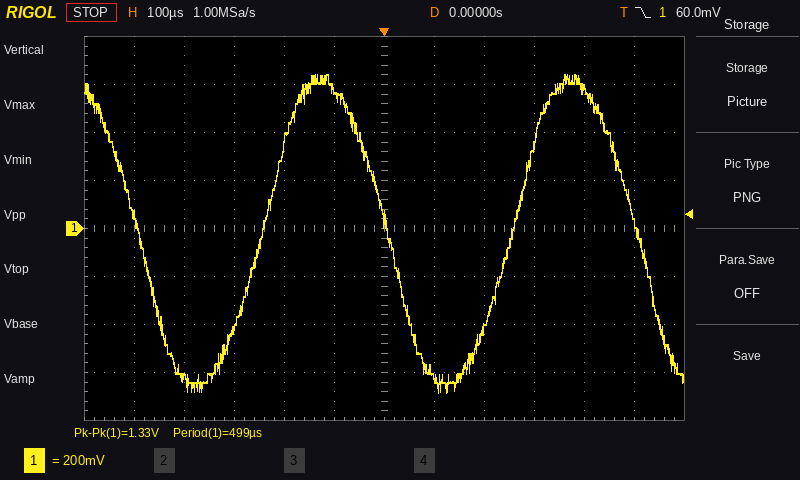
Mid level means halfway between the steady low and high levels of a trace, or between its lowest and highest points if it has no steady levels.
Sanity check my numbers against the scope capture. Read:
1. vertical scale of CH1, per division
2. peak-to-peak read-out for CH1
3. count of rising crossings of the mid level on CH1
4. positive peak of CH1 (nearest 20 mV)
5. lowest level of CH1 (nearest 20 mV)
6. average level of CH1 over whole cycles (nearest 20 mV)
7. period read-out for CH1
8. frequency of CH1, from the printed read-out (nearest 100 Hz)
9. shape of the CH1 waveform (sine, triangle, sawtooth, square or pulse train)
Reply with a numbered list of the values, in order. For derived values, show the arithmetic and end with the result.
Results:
1. 200 mV
2. 1.33 V
3. 2
4. 640 mV
5. -680 mV
6. (640 mV + (-680 mV)) / 2 ≈ -20 mV
7. 499 µs
8. 1 / 499 µs ≈ 2.0 kHz
9. sine
